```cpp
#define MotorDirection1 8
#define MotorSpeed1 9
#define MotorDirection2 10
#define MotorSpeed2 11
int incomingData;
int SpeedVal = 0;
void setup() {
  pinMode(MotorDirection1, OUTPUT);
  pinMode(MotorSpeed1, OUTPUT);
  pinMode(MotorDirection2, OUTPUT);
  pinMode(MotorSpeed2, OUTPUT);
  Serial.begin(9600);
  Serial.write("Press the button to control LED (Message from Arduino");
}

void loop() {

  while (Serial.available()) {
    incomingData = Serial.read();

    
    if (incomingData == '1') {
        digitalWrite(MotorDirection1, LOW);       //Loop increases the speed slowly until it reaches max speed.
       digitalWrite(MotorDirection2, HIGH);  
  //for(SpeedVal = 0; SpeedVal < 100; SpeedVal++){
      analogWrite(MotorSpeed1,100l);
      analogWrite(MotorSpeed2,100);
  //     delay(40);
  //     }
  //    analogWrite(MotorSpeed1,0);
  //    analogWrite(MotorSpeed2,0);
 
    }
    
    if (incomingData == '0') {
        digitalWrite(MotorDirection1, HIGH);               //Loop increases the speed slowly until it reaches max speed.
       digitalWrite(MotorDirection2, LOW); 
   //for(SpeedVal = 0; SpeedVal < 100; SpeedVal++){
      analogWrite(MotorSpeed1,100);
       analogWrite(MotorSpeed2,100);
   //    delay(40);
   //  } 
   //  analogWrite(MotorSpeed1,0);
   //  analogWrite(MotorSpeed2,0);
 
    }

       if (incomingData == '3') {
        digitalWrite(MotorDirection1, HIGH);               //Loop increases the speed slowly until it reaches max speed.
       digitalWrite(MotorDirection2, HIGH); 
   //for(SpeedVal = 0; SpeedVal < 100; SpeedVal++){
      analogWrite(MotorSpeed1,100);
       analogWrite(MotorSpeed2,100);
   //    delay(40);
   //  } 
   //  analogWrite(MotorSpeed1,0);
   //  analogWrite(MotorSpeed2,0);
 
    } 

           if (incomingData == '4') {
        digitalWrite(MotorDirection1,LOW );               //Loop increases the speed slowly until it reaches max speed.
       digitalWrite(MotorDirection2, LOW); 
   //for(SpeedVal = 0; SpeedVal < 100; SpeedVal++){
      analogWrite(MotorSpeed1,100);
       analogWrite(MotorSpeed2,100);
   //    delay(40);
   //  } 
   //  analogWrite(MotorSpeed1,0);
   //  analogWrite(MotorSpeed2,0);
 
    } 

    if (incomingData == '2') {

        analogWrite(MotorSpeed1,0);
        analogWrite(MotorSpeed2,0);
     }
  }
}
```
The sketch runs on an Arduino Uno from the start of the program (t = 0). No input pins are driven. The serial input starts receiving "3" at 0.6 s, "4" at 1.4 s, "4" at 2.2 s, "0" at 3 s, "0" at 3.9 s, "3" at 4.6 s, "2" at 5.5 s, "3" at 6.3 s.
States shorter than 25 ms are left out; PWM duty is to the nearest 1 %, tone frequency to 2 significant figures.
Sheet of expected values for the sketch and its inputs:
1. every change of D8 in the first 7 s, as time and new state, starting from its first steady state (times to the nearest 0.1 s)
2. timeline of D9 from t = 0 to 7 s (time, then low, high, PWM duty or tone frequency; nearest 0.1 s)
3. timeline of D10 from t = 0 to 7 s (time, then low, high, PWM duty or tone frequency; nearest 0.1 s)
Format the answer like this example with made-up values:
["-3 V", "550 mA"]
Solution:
["0 s low; 0.6 s high; 1.4 s low; 3 s high", "0 s low; 0.6 s PWM 39 %; 5.5 s low; 6.3 s PWM 39 %", "0 s low; 0.6 s high; 1.4 s low; 4.6 s high"]
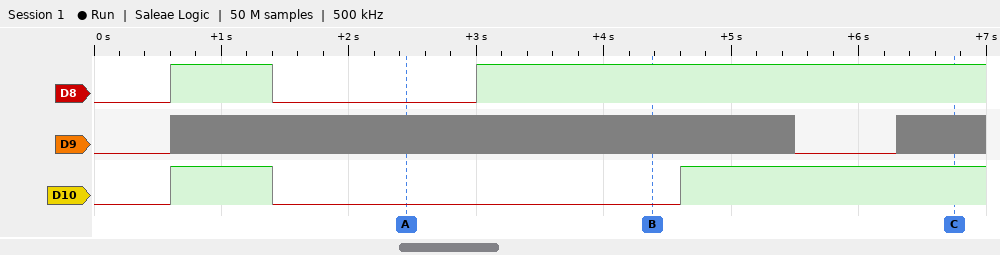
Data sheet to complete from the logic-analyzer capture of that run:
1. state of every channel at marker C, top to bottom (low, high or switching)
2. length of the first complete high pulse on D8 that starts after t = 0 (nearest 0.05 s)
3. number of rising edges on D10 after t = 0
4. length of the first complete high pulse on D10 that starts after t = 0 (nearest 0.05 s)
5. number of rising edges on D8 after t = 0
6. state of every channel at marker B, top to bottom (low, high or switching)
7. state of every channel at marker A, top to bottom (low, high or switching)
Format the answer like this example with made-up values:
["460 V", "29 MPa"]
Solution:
["D8 high, D9 switching, D10 high", "0.80 s", "2", "0.80 s", "2", "D8 high, D9 switching, D10 low", "D8 low, D9 switching, D10 low"]
